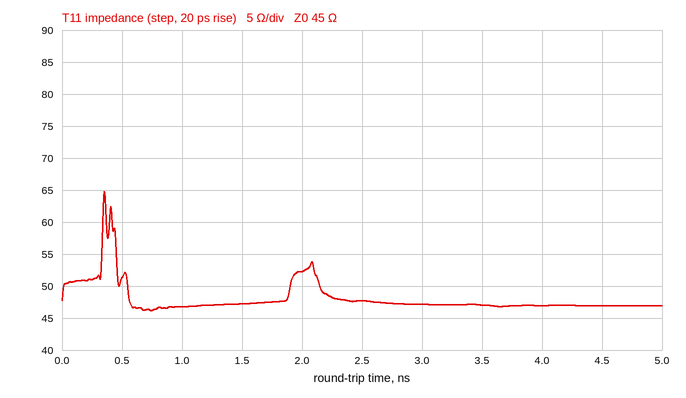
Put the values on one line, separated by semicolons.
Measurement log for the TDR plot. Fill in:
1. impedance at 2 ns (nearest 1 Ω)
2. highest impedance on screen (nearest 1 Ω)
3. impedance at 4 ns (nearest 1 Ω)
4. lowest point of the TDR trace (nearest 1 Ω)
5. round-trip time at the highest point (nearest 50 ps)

52 Ω; 65 Ω; 47 Ω; 46 Ω; 350 ps
